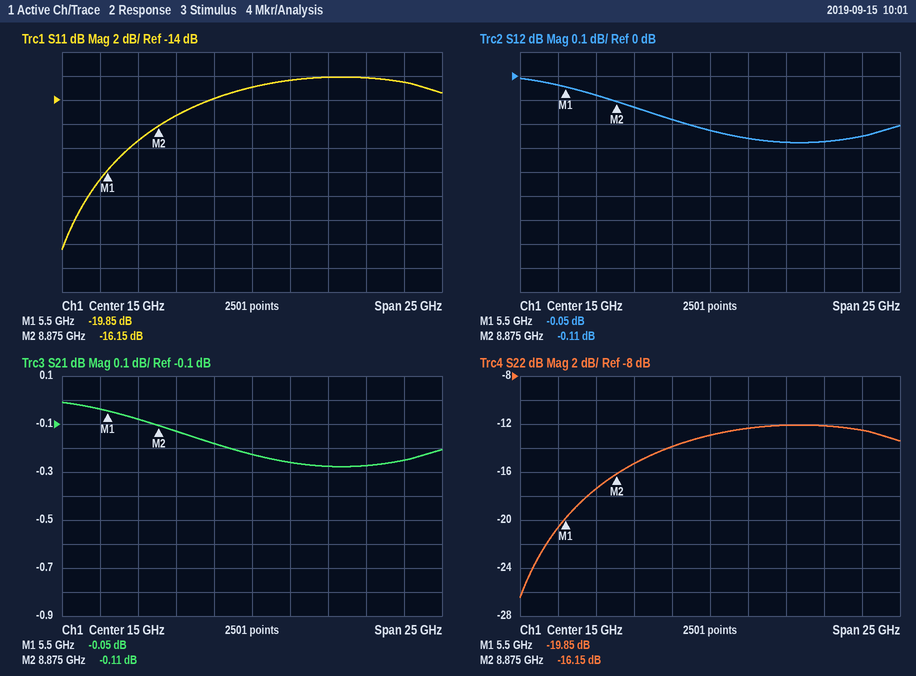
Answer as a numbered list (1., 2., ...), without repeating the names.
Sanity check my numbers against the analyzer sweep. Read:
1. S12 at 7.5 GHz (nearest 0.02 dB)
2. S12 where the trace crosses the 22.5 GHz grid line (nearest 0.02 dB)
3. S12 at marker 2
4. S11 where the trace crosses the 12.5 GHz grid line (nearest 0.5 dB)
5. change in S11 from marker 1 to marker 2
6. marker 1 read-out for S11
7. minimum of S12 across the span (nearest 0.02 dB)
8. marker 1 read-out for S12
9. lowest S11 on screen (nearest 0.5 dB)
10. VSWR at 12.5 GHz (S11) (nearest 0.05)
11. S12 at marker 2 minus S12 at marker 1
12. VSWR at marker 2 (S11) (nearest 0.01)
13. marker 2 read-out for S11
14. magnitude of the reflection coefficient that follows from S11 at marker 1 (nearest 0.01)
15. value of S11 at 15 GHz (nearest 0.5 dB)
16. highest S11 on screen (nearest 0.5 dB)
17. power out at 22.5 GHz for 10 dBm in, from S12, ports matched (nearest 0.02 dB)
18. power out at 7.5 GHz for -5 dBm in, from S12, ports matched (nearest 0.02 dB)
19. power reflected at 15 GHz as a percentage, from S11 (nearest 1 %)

1. -0.08 dB
2. -0.28 dB
3. -0.11 dB
4. -14.0 dB
5. 3.70 dB
6. -19.85 dB
7. -0.28 dB
8. -0.05 dB
9. -26.5 dB
10. 1.50
11. -0.06 dB
12. 1.37
13. -16.15 dB
14. 0.10
15. -13.0 dB
16. -12.0 dB
17. 9.72 dBm
18. -5.08 dBm
19. 5 %
